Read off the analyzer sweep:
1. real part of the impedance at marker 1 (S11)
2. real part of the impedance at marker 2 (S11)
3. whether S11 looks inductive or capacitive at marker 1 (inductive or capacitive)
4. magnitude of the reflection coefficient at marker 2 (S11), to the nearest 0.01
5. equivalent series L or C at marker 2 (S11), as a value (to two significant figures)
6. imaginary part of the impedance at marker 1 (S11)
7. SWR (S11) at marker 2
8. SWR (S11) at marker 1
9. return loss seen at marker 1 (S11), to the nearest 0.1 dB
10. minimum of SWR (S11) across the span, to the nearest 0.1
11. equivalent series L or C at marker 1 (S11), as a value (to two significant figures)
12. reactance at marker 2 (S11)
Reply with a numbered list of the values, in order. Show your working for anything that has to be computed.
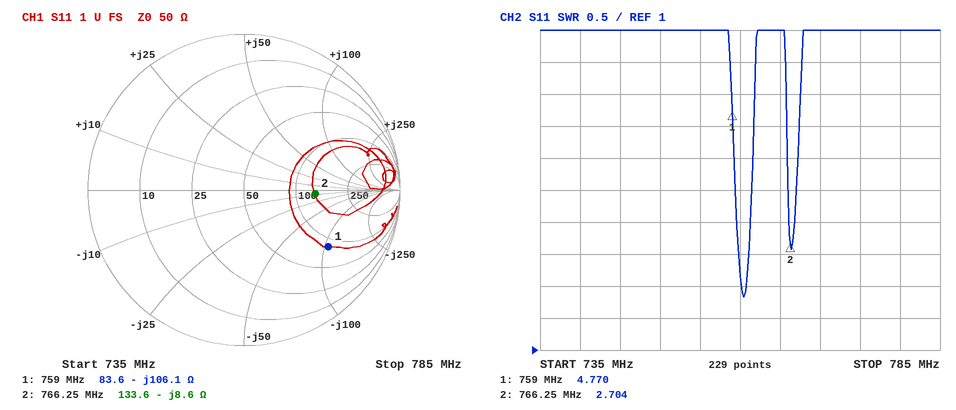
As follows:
1. 83.6 Ω
2. 133.6 Ω
3. capacitive
4. 0.46
5. C = 1/(2π × 766.25 MHz × 8.6 Ω) ≈ 24 pF
6. -106.1 Ω
7. 2.704
8. 4.770
9. 3.7 dB
10. 1.8
11. C = 1/(2π × 759 MHz × 106.1 Ω) ≈ 2.0 pF
12. -8.6 Ω
